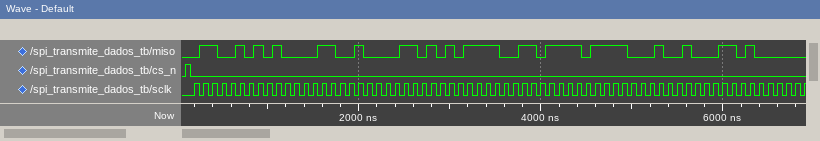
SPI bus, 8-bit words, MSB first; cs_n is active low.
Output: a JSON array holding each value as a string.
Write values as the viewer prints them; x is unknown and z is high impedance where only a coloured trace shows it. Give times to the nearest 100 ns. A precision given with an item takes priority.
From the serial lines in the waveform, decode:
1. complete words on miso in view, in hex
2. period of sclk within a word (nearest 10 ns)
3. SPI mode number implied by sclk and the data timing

["65, 43, 21, AB, CD, EF, 12, 34", "100 ns", "0"]
